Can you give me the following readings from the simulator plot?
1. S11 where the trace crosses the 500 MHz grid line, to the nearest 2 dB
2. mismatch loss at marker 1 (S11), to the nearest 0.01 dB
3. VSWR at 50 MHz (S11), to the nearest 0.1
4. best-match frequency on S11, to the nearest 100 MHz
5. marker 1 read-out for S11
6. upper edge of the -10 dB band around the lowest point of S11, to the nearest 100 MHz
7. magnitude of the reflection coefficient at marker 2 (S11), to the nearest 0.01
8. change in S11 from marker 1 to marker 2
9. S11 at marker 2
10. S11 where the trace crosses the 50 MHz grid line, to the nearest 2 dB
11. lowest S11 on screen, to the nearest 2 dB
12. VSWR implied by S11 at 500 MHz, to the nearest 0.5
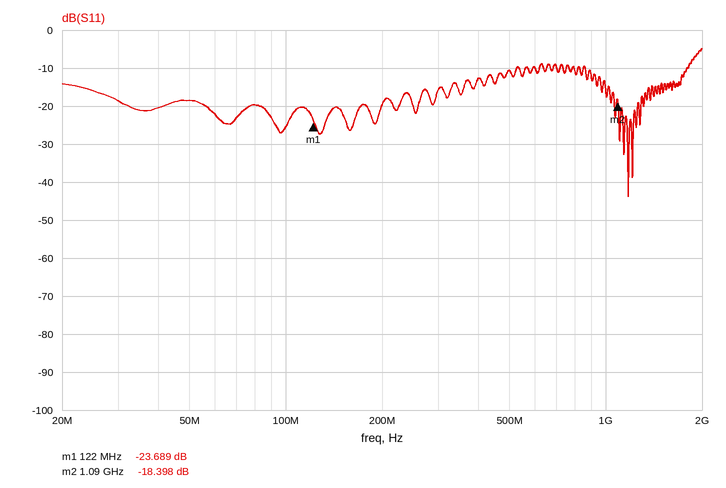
-10 dB
0.02 dB
1.3
1.2 GHz
-23.689 dB
1.8 GHz
0.12
5.291 dB
-18.398 dB
-18 dB
-44 dB
2.0
